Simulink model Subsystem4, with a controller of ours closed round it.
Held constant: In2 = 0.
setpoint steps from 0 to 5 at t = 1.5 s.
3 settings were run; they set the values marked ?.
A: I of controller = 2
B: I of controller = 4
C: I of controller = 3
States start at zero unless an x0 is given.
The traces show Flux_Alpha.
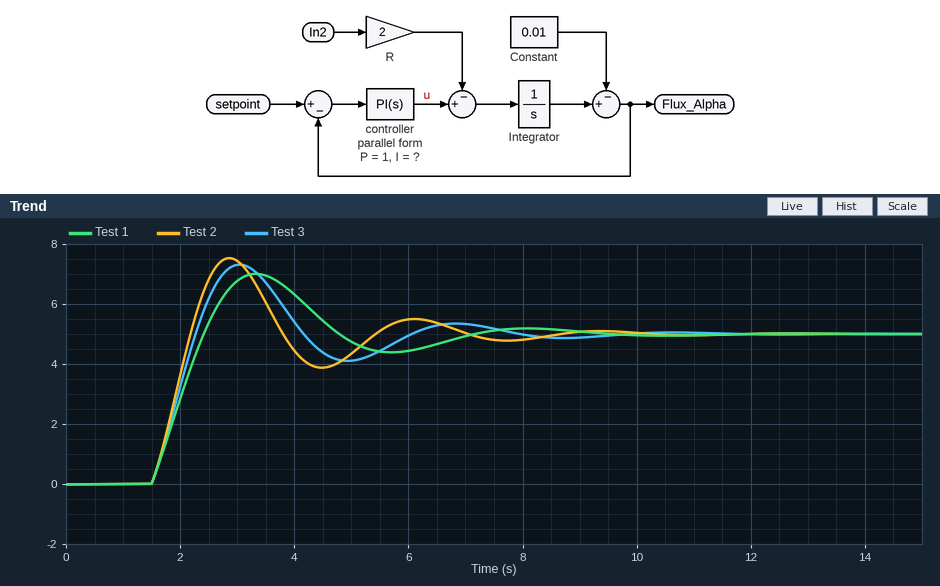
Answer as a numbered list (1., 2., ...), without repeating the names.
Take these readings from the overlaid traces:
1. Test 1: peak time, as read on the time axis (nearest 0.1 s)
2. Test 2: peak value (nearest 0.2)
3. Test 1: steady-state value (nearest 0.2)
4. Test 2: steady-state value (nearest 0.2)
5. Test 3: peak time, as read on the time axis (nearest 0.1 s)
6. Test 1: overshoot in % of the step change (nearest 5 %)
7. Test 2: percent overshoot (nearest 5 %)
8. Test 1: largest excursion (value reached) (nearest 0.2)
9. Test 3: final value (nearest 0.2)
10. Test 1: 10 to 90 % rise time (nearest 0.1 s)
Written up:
1. 3.3 s
2. 7.6
3. 5.0
4. 5.0
5. 3.0 s
6. 40 %
7. 50 %
8. 7.0
9. 5.0
10. 0.7 s
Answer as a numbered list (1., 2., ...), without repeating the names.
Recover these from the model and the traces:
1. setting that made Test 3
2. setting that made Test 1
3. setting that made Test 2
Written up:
1. C
2. A
3. B
